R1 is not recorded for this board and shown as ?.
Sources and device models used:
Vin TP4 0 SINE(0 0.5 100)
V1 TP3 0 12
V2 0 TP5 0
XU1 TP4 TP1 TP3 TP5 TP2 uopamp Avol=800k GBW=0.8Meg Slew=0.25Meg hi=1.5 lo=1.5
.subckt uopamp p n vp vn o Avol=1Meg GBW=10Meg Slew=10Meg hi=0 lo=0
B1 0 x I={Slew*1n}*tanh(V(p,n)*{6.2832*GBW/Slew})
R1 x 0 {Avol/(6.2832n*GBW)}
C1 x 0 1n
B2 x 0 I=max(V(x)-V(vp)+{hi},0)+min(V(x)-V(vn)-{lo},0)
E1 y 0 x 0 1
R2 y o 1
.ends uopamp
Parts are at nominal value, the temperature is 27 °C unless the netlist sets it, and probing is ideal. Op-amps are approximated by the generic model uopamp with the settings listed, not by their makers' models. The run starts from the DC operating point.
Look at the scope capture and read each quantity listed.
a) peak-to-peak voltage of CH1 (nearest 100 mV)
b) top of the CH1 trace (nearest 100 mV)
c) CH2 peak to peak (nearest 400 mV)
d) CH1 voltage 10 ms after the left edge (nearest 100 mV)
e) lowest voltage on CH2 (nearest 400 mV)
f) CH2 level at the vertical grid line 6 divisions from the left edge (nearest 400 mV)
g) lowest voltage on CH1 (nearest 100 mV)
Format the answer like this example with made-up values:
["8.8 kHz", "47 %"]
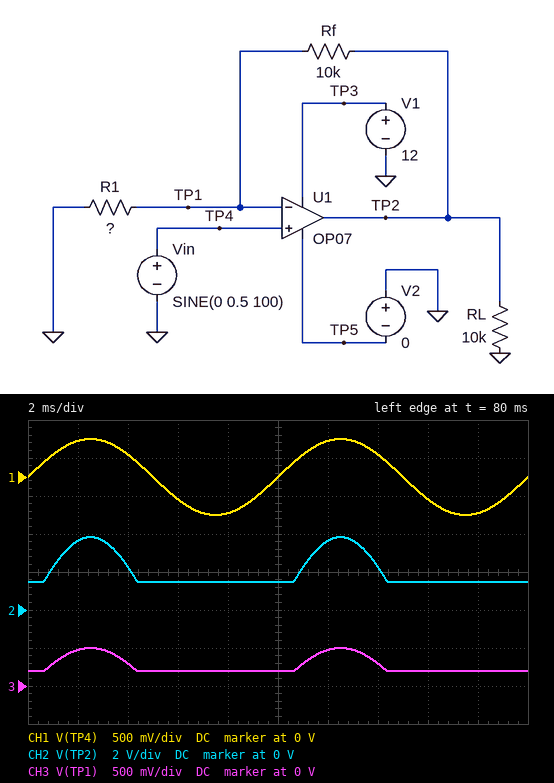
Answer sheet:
["1.0 V", "500 mV", "2.4 V", "0 V", "1.6 V", "3.6 V", "-500 mV"]
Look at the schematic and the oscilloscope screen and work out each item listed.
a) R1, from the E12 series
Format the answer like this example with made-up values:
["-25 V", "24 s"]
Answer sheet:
["1.5 kΩ"]
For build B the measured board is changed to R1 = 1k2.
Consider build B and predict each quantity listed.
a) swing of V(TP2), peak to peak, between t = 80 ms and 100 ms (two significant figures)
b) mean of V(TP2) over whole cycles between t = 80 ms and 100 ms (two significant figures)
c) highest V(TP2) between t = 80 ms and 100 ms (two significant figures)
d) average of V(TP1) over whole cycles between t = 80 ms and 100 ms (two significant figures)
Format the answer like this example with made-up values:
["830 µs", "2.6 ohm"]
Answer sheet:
["3.2 V", "2.3 V", "4.7 V", "250 mV"]
